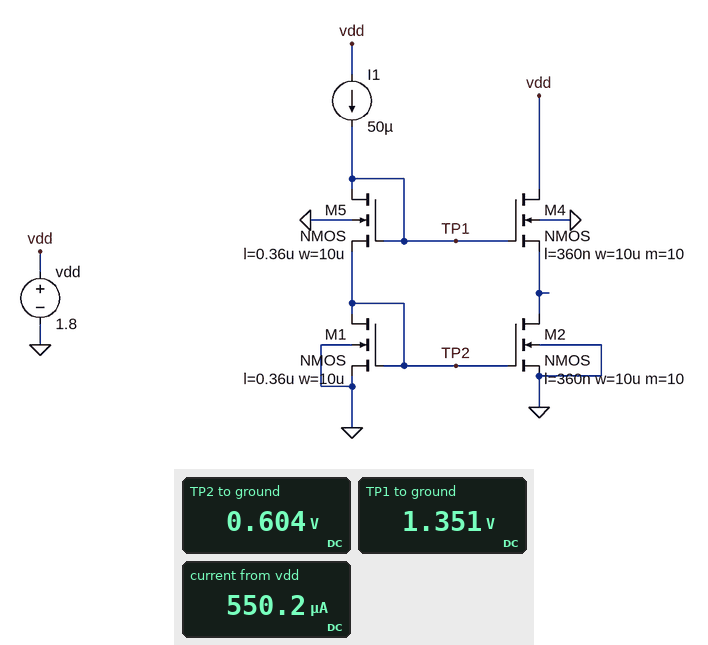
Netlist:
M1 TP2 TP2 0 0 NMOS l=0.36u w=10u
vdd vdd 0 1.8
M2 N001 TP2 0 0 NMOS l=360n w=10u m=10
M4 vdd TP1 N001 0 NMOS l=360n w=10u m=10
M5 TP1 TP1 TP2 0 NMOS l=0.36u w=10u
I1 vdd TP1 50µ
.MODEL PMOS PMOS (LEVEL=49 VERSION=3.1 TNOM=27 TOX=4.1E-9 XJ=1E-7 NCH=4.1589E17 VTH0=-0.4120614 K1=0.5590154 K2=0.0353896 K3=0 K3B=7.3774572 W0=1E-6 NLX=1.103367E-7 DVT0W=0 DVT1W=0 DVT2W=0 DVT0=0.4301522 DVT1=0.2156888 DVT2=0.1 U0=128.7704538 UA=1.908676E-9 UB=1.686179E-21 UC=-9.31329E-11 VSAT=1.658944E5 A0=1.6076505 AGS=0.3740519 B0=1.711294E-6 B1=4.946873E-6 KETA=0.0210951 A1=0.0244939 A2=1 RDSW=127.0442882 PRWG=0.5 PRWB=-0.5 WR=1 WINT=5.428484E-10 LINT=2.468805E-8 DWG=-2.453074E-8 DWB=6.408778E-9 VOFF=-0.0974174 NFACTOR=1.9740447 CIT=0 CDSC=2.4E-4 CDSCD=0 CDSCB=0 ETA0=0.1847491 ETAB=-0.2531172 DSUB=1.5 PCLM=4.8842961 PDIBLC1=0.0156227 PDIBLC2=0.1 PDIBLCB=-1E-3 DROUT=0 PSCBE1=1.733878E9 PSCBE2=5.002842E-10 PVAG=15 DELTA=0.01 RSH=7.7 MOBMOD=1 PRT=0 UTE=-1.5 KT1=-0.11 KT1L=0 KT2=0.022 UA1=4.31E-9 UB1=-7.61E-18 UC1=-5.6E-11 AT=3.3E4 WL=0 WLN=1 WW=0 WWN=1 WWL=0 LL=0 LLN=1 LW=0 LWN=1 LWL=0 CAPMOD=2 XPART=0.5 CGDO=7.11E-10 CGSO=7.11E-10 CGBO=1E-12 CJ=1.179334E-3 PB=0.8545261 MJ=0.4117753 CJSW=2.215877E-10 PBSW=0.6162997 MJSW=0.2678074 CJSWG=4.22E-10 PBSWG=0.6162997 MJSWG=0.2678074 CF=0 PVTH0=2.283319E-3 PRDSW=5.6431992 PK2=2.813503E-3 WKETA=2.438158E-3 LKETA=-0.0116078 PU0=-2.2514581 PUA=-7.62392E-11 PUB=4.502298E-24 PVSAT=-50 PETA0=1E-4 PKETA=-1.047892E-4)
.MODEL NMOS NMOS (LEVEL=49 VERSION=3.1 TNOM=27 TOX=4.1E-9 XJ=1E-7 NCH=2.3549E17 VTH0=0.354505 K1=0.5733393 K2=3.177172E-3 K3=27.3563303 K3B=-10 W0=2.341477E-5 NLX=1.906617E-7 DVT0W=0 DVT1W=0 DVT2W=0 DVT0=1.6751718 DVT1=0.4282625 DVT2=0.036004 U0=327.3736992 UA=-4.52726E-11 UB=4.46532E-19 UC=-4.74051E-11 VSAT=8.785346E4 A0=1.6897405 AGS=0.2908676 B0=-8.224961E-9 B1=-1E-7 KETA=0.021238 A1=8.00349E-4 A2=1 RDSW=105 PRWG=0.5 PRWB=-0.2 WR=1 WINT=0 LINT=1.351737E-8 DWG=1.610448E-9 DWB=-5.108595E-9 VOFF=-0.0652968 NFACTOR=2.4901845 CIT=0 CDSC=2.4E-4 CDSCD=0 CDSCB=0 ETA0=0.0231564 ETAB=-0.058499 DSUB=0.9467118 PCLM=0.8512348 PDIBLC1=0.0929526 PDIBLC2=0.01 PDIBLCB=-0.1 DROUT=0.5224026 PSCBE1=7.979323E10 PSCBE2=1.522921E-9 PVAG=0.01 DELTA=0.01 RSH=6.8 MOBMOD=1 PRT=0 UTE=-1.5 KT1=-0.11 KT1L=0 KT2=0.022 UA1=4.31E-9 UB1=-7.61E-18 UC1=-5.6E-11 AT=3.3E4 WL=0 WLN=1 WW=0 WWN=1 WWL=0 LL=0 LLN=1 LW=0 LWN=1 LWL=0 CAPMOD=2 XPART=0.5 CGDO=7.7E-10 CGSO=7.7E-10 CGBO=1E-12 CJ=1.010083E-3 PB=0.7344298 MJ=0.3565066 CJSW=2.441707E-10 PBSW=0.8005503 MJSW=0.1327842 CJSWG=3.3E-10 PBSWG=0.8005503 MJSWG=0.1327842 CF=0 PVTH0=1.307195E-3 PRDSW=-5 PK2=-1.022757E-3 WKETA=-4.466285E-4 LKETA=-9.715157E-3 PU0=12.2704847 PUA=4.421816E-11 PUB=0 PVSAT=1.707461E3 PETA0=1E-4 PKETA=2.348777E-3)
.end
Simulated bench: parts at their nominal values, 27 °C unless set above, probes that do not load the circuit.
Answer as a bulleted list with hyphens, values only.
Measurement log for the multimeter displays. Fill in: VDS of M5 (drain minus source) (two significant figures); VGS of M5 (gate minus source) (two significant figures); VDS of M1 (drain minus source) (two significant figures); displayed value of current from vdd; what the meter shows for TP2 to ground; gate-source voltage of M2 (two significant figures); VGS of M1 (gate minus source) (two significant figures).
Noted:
- 750 mV
- 750 mV
- 600 mV
- 550.2 µA
- 0.604 V
- 600 mV
- 600 mV
